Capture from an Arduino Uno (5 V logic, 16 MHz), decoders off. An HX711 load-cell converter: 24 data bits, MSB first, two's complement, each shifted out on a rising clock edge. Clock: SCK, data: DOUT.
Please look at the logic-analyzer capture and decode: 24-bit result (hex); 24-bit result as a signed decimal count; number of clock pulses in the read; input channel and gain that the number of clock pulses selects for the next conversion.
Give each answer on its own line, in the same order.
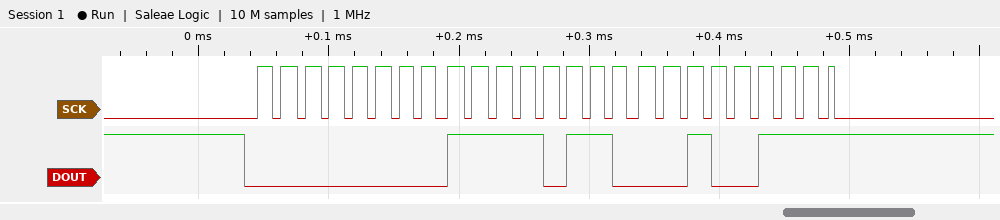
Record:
0x00F627
63015
25
channel A, gain 128
